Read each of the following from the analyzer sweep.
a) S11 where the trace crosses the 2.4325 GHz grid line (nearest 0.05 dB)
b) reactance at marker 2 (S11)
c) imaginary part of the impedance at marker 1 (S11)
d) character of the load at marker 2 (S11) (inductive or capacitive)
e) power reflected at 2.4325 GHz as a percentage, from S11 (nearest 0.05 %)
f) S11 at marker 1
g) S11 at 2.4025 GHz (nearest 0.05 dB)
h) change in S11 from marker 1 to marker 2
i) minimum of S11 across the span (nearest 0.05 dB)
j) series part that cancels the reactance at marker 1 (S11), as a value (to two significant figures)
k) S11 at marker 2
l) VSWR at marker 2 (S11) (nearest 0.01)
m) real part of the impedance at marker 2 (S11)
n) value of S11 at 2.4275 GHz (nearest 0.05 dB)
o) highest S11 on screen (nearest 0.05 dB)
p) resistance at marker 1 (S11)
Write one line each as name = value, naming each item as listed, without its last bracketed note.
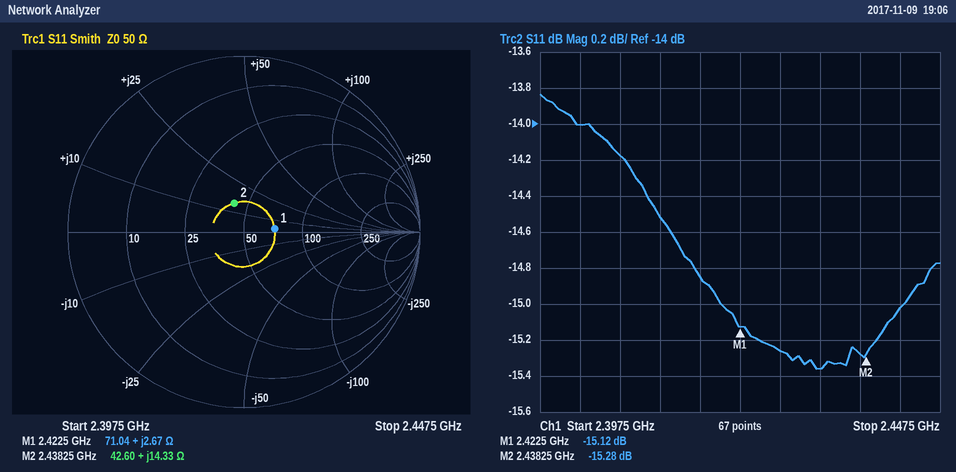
S11 where the trace crosses the 2.4325 GHz grid line = -15.35 dB
reactance at marker 2 = +14.33 Ω
imaginary part of the impedance at marker 1 = +2.67 Ω
character of the load at marker 2 (S11) = inductive
power reflected at 2.4325 GHz as a percentage, from S11 = 2.90 %
S11 at marker 1 = -15.12 dB
S11 at 2.4025 GHz = -14.00 dB
change in S11 from marker 1 to marker 2 = -0.16 dB
minimum of S11 across the span = -15.35 dB
series part that cancels the reactance at marker 1 (S11), as a value = 25 pF
S11 at marker 2 = -15.28 dB
VSWR at marker 2 (S11) = 1.42
real part of the impedance at marker 2 = 42.60 Ω
value of S11 at 2.4275 GHz = -15.25 dB
highest S11 on screen = -13.85 dB
resistance at marker 1 = 71.04 Ω
